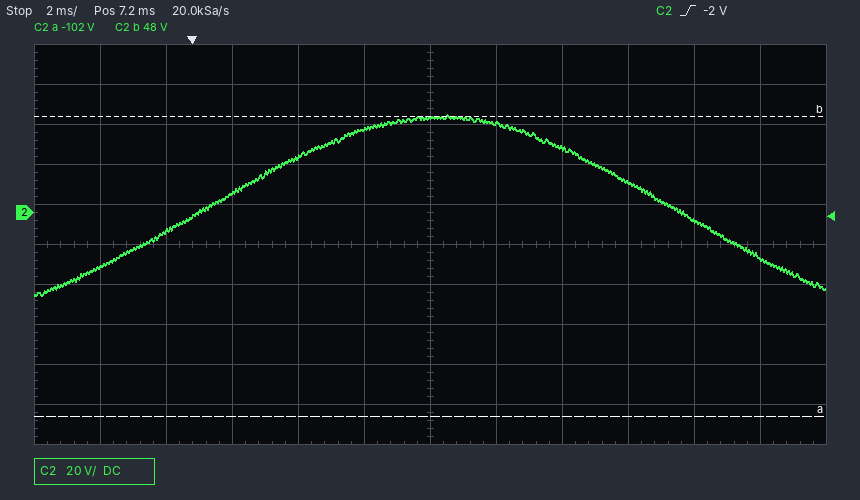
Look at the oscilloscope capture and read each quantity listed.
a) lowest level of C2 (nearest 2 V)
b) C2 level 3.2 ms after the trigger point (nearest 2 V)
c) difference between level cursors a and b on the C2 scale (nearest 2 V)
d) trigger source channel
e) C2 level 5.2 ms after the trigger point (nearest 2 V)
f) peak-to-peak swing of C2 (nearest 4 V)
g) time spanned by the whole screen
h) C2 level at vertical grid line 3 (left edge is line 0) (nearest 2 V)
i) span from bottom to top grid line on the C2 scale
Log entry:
-42 V
28 V
150 V
C2
42 V
92 V
24 ms
10 V
200 V
